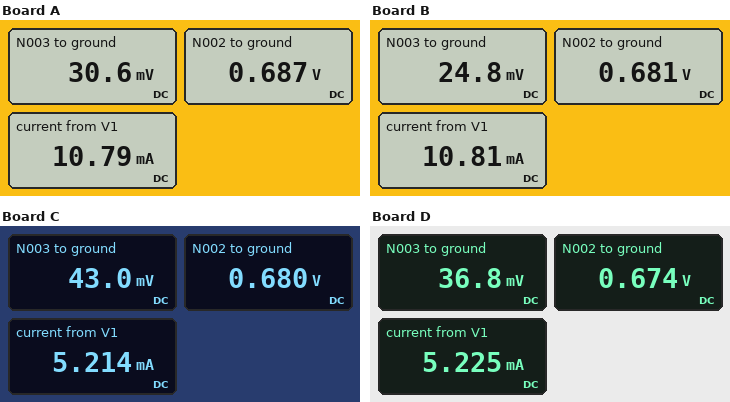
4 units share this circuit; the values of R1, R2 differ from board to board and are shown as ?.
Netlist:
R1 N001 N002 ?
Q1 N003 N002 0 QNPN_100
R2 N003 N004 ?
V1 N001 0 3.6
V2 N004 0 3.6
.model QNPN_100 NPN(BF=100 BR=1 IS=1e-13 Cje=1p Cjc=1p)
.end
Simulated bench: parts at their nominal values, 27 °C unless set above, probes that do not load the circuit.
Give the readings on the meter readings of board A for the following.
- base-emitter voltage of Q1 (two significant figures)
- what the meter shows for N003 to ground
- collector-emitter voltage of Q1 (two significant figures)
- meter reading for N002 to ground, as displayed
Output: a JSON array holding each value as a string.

["690 mV", "30.6 mV", "31 mV", "0.687 V"]
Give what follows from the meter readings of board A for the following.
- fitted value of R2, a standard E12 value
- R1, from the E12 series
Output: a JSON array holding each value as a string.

["270 Ω", "270 Ω"]
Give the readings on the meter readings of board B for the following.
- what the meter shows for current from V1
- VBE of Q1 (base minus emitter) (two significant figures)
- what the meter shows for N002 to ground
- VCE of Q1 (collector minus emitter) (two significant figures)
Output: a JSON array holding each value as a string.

["10.81 mA", "680 mV", "0.681 V", "25 mV"]
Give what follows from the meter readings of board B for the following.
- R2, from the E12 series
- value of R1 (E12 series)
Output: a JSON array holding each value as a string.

["560 Ω", "270 Ω"]
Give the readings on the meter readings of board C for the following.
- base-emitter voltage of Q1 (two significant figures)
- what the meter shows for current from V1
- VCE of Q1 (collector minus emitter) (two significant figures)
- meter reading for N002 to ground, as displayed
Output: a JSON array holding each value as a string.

["680 mV", "5.214 mA", "43 mV", "0.680 V"]
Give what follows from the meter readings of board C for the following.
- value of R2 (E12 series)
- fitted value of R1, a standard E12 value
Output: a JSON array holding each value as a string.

["220 Ω", "560 Ω"]
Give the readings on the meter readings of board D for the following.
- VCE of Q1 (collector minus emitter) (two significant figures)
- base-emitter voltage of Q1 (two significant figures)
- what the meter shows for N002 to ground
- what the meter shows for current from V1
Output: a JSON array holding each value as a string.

["37 mV", "670 mV", "0.674 V", "5.225 mA"]
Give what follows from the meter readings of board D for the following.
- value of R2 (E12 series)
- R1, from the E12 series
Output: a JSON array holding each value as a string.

["330 Ω", "560 Ω"]
